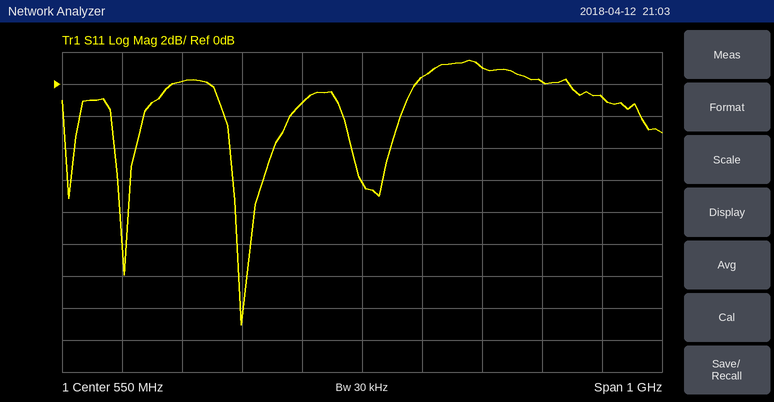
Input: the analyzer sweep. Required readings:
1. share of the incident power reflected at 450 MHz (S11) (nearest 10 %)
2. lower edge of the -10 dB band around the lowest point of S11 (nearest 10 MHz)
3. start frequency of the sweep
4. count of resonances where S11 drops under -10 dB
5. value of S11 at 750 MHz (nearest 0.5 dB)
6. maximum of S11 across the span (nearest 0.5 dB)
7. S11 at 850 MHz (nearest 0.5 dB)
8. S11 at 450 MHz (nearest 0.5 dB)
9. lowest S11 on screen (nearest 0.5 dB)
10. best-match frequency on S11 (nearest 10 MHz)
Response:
80 %
340 MHz
50 MHz
2
1.0 dB
1.5 dB
0.0 dB
-1.0 dB
-15.0 dB
350 MHz
